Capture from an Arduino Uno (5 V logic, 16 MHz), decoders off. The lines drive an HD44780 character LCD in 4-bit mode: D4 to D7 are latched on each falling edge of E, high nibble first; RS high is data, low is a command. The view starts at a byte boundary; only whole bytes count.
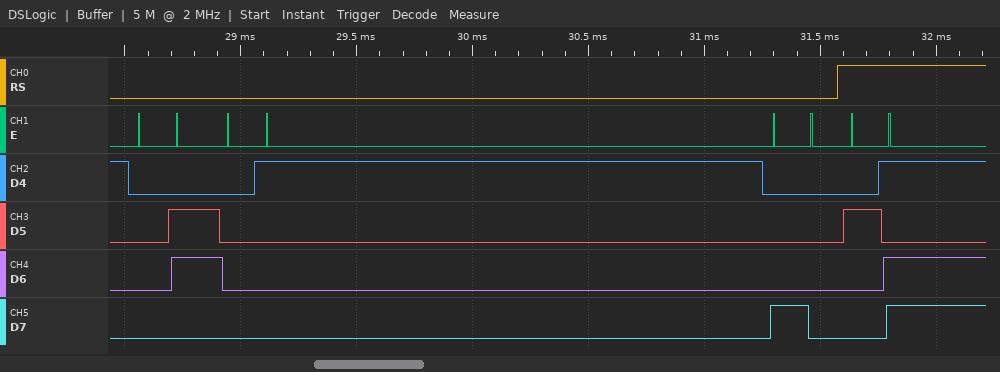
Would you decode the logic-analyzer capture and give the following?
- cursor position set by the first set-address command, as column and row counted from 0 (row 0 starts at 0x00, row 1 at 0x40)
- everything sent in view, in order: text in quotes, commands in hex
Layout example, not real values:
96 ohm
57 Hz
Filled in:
column 0, row 0
0x06 0x01 0x80 "-"
